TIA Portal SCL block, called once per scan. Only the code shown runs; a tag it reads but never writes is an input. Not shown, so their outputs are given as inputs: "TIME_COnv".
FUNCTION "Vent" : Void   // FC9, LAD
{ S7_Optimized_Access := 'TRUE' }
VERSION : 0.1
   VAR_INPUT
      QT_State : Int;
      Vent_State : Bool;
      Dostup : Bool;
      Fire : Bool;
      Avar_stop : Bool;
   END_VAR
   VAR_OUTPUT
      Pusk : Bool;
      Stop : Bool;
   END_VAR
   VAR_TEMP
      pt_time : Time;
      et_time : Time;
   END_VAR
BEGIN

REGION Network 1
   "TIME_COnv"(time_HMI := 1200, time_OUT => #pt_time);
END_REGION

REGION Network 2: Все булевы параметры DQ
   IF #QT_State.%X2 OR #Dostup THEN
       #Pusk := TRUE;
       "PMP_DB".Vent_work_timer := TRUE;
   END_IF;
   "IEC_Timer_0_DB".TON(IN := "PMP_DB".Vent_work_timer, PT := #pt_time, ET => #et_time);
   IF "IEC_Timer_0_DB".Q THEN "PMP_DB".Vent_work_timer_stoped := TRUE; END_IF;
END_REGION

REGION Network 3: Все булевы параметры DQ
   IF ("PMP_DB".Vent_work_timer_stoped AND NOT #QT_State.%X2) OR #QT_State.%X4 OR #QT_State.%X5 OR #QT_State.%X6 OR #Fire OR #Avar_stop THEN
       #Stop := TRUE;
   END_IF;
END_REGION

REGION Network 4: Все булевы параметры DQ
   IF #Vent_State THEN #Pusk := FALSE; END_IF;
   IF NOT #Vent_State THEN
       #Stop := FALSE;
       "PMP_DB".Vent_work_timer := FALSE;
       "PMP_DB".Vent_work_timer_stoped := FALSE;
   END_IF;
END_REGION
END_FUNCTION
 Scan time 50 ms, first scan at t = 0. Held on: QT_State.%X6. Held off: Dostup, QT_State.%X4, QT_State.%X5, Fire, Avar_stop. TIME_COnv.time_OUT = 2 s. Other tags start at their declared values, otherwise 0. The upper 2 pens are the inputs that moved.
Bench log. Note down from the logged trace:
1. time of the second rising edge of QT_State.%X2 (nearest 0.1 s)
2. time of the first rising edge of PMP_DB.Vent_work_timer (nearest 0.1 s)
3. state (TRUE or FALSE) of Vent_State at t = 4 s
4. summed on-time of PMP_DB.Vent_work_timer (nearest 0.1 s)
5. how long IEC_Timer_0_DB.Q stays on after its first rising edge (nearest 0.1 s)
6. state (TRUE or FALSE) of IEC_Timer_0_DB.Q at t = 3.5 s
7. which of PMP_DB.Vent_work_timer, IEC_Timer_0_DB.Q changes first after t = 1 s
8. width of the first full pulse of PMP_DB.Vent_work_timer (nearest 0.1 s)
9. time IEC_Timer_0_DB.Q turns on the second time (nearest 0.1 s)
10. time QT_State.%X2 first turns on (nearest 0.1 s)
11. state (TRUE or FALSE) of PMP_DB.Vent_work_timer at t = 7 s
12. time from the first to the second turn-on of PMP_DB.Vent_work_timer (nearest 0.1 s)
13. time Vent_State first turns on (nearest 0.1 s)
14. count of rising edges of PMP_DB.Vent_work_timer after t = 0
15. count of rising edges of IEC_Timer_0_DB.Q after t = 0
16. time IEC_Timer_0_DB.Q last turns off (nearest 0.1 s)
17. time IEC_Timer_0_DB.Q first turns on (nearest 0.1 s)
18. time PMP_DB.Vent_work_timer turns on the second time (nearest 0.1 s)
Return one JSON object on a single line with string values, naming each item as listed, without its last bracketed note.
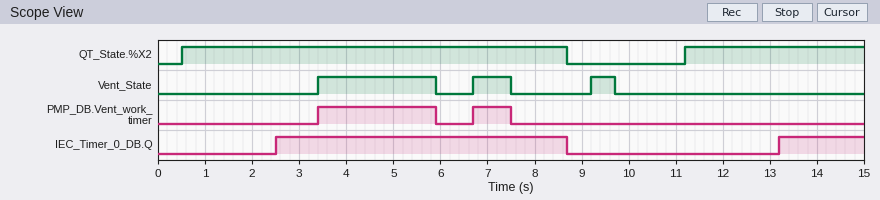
{"time of the second rising edge of QT_State.%X2": "11.2 s", "time of the first rising edge of PMP_DB.Vent_work_timer": "3.4 s", "state (TRUE or FALSE) of Vent_State at t = 4 s": "TRUE", "summed on-time of PMP_DB.Vent_work_timer": "3.3 s", "how long IEC_Timer_0_DB.Q stays on after its first rising edge": "6.2 s", "state (TRUE or FALSE) of IEC_Timer_0_DB.Q at t = 3.5 s": "TRUE", "which of PMP_DB.Vent_work_timer, IEC_Timer_0_DB.Q changes first after t = 1 s": "IEC_Timer_0_DB.Q", "width of the first full pulse of PMP_DB.Vent_work_timer": "2.5 s", "time IEC_Timer_0_DB.Q turns on the second time": "13.2 s", "time QT_State.%X2 first turns on": "0.5 s", "state (TRUE or FALSE) of PMP_DB.Vent_work_timer at t = 7 s": "TRUE", "time from the first to the second turn-on of PMP_DB.Vent_work_timer": "3.3 s", "time Vent_State first turns on": "3.4 s", "count of rising edges of PMP_DB.Vent_work_timer after t = 0": "2", "count of rising edges of IEC_Timer_0_DB.Q after t = 0": "2", "time IEC_Timer_0_DB.Q last turns off": "8.7 s", "time IEC_Timer_0_DB.Q first turns on": "2.5 s", "time PMP_DB.Vent_work_timer turns on the second time": "6.7 s"}
